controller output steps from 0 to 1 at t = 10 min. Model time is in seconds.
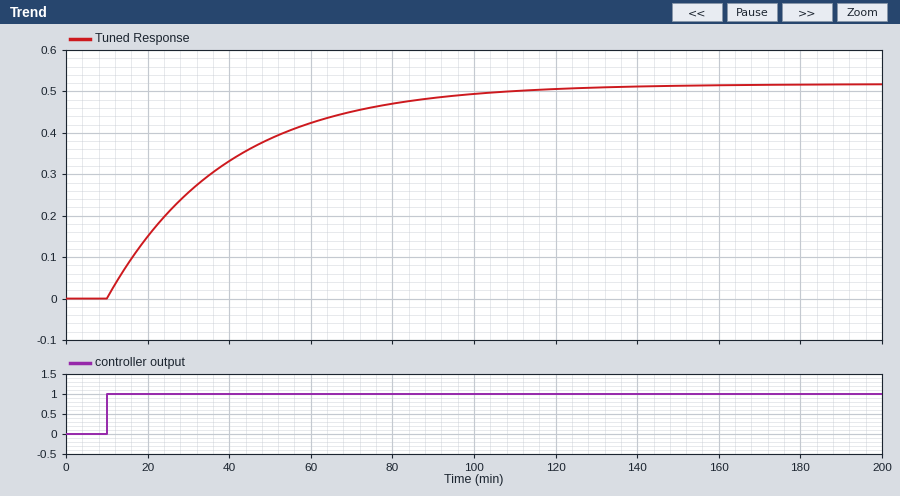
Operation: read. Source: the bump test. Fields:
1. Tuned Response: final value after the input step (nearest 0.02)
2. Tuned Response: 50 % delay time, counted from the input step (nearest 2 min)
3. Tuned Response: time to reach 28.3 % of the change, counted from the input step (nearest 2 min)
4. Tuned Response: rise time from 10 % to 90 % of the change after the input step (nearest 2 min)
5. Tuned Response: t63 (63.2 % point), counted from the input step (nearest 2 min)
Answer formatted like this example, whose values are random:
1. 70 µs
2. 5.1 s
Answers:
1. 0.52
2. 20 min
3. 10 min
4. 64 min
5. 30 min
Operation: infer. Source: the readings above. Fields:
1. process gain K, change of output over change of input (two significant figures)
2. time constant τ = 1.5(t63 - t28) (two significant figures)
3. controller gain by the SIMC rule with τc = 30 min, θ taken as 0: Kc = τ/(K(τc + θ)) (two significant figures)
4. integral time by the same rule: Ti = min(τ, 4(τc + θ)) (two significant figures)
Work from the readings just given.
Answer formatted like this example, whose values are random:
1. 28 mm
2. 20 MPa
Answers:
1. 0.52
2. 30 min
3. 1.9
4. 30 min
